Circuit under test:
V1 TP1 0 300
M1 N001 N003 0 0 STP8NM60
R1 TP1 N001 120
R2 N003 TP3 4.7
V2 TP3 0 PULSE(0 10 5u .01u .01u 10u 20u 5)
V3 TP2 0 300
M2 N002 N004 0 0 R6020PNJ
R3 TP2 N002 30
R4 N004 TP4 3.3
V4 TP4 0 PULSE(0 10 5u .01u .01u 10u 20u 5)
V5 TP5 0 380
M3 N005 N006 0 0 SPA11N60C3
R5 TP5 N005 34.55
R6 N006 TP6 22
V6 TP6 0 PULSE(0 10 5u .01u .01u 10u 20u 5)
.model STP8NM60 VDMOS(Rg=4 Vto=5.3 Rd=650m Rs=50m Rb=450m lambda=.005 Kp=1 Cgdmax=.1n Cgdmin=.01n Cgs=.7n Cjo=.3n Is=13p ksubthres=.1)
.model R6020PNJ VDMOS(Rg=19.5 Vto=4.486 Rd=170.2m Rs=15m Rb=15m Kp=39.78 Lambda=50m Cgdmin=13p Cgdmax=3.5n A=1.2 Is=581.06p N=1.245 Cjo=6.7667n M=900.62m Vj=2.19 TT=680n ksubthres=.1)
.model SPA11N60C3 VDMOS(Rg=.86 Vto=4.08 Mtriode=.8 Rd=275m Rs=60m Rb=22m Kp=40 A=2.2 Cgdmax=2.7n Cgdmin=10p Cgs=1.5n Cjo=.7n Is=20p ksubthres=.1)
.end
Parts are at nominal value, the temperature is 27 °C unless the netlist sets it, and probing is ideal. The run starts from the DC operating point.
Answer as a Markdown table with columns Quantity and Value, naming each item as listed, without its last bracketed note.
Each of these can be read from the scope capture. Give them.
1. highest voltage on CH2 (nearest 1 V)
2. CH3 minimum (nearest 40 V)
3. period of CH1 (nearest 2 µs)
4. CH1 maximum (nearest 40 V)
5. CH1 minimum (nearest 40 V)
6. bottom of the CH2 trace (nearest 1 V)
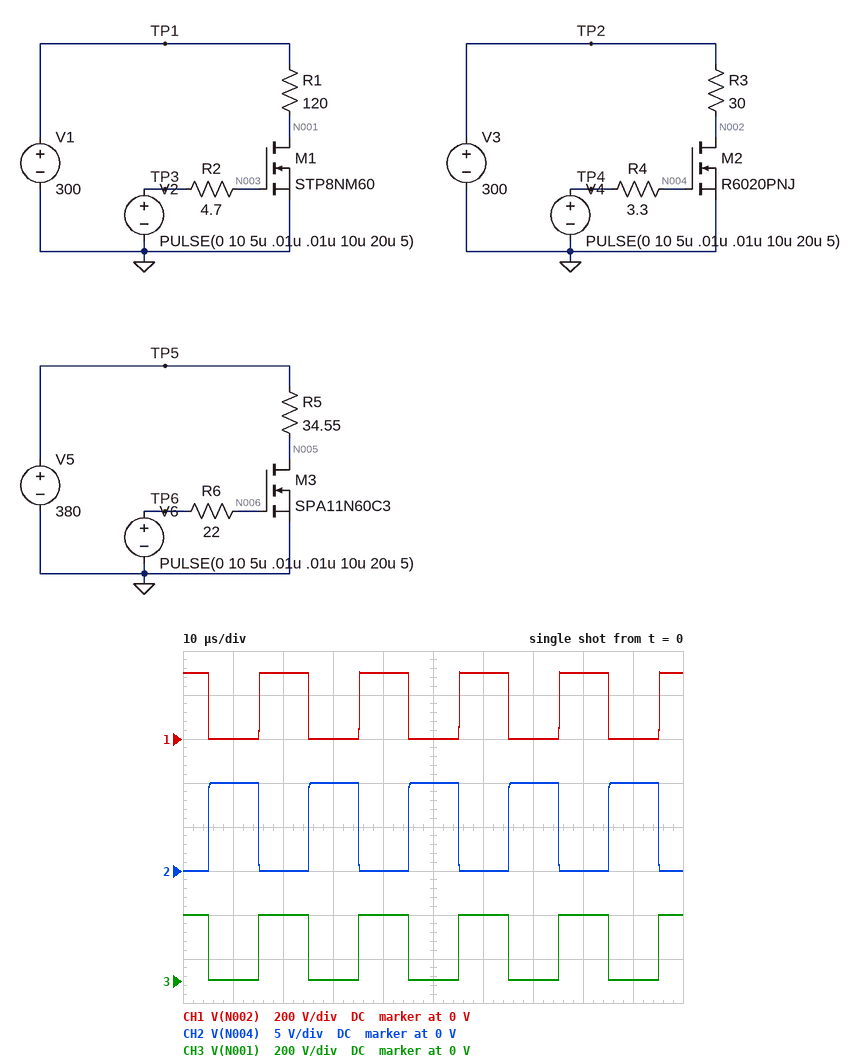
| Quantity | Value |
|---|---|
| highest voltage on CH2 | 10 V |
| CH3 minimum | 0 V |
| period of CH1 | 20 µs |
| CH1 maximum | 320 V |
| CH1 minimum | 0 V |
| bottom of the CH2 trace | 0 V |
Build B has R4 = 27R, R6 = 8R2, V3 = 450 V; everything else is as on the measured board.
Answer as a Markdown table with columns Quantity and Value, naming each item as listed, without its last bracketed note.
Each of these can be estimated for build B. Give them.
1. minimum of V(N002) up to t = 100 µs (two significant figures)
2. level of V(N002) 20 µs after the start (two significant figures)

| Quantity | Value |
|---|---|
| minimum of V(N002) up to t = 100 µs | 2.8 V |
| level of V(N002) 20 µs after the start | 450 V |
